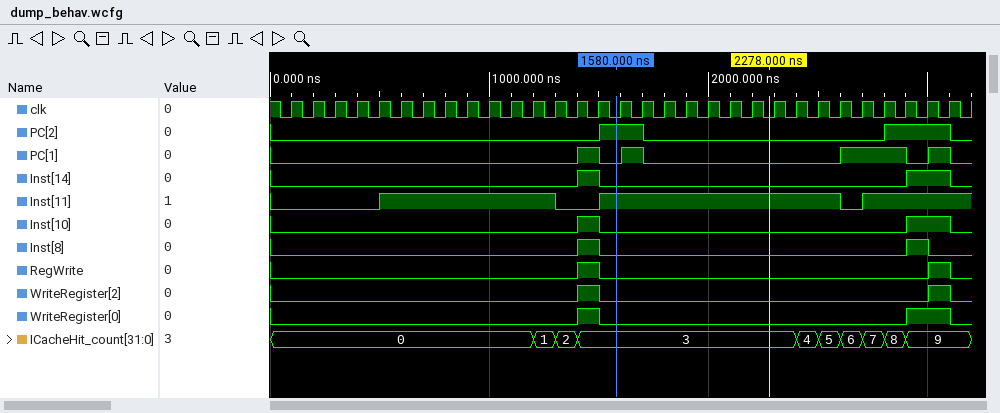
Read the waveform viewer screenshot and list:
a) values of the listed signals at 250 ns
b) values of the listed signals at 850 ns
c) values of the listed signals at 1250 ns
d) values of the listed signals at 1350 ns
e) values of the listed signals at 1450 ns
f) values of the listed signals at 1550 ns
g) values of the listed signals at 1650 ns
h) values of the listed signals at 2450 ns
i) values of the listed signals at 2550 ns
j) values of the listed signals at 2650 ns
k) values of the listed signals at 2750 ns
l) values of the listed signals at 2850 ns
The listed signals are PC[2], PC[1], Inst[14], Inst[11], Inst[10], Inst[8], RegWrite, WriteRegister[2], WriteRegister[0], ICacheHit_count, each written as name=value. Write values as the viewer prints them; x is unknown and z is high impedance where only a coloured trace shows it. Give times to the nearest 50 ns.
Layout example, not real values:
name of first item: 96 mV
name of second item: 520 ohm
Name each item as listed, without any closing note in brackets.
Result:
values of the listed signals at 250 ns: PC[2]=0, PC[1]=0, Inst[14]=0, Inst[11]=0, Inst[10]=0, Inst[8]=0, RegWrite=0, WriteRegister[2]=0, WriteRegister[0]=0, ICacheHit_count=0
values of the listed signals at 850 ns: PC[2]=0, PC[1]=0, Inst[14]=0, Inst[11]=1, Inst[10]=0, Inst[8]=0, RegWrite=0, WriteRegister[2]=0, WriteRegister[0]=0, ICacheHit_count=0
values of the listed signals at 1250 ns: PC[2]=0, PC[1]=0, Inst[14]=0, Inst[11]=1, Inst[10]=0, Inst[8]=0, RegWrite=0, WriteRegister[2]=0, WriteRegister[0]=0, ICacheHit_count=1
values of the listed signals at 1350 ns: PC[2]=0, PC[1]=0, Inst[14]=0, Inst[11]=0, Inst[10]=0, Inst[8]=0, RegWrite=0, WriteRegister[2]=0, WriteRegister[0]=0, ICacheHit_count=2
values of the listed signals at 1450 ns: PC[2]=0, PC[1]=1, Inst[14]=1, Inst[11]=0, Inst[10]=1, Inst[8]=1, RegWrite=1, WriteRegister[2]=1, WriteRegister[0]=1, ICacheHit_count=3
values of the listed signals at 1550 ns: PC[2]=1, PC[1]=0, Inst[14]=0, Inst[11]=1, Inst[10]=0, Inst[8]=0, RegWrite=0, WriteRegister[2]=0, WriteRegister[0]=0, ICacheHit_count=3
values of the listed signals at 1650 ns: PC[2]=1, PC[1]=1, Inst[14]=0, Inst[11]=1, Inst[10]=0, Inst[8]=0, RegWrite=0, WriteRegister[2]=0, WriteRegister[0]=0, ICacheHit_count=3
values of the listed signals at 2450 ns: PC[2]=0, PC[1]=0, Inst[14]=0, Inst[11]=1, Inst[10]=0, Inst[8]=0, RegWrite=0, WriteRegister[2]=0, WriteRegister[0]=0, ICacheHit_count=4
values of the listed signals at 2550 ns: PC[2]=0, PC[1]=0, Inst[14]=0, Inst[11]=1, Inst[10]=0, Inst[8]=0, RegWrite=0, WriteRegister[2]=0, WriteRegister[0]=0, ICacheHit_count=5
values of the listed signals at 2650 ns: PC[2]=0, PC[1]=1, Inst[14]=0, Inst[11]=0, Inst[10]=0, Inst[8]=0, RegWrite=0, WriteRegister[2]=0, WriteRegister[0]=0, ICacheHit_count=6
values of the listed signals at 2750 ns: PC[2]=0, PC[1]=1, Inst[14]=0, Inst[11]=1, Inst[10]=0, Inst[8]=0, RegWrite=0, WriteRegister[2]=0, WriteRegister[0]=0, ICacheHit_count=7
values of the listed signals at 2850 ns: PC[2]=1, PC[1]=1, Inst[14]=0, Inst[11]=1, Inst[10]=0, Inst[8]=0, RegWrite=0, WriteRegister[2]=0, WriteRegister[0]=0, ICacheHit_count=8
